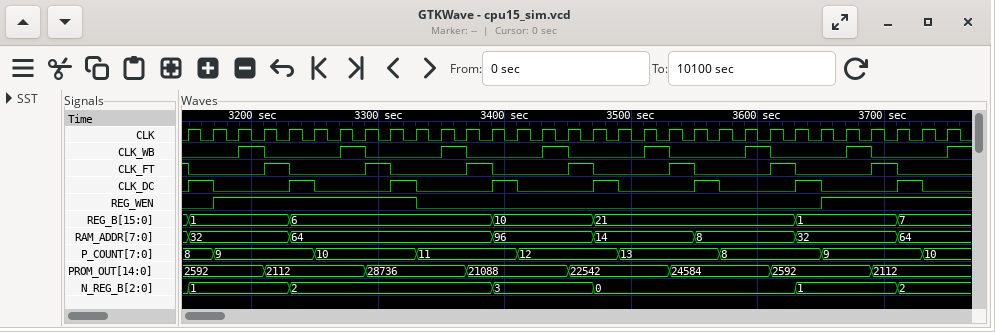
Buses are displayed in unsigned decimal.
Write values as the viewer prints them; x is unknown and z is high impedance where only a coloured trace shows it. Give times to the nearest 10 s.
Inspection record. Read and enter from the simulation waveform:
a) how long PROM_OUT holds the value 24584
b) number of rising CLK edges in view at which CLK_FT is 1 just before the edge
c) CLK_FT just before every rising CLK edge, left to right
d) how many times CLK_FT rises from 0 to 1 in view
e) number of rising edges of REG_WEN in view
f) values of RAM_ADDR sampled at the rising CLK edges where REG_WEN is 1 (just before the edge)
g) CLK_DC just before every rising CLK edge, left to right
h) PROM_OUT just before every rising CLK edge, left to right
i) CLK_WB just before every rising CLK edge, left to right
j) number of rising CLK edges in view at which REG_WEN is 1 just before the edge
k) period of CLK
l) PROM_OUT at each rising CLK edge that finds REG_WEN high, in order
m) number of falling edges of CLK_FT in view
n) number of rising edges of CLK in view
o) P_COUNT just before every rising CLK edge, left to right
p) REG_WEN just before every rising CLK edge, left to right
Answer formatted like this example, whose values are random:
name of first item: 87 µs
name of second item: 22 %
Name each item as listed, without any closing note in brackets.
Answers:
how long PROM_OUT holds the value 24584: 80 s
number of rising CLK edges in view at which CLK_FT is 1 just before the edge: 8
CLK_FT just before every rising CLK edge, left to right: 1 0 0 0 1 0 0 0 1 0 0 0 1 0 0 0 1 0 0 0 1 0 0 0 1 0 0 0 1 0 0
how many times CLK_FT rises from 0 to 1 in view: 7
number of rising edges of REG_WEN in view: 2
values of RAM_ADDR sampled at the rising CLK edges where REG_WEN is 1: 32, 32, 32, 64, 64, 64, 64, 64, 32, 32, 32, 64, 64
CLK_DC just before every rising CLK edge, left to right: 0 1 0 0 0 1 0 0 0 1 0 0 0 1 0 0 0 1 0 0 0 1 0 0 0 1 0 0 0 1 0
PROM_OUT just before every rising CLK edge, left to right: 2592, 2592, 2592, 2592, 2112, 2112, 2112, 2112, 28736, 28736, 28736, 28736, 21088, 21088, 21088, 21088, 22542, 22542, 22542, 22542, 24584, 24584, 24584, 24584, 2592, 2592, 2592, 2592, 2112, 2112, 2112
CLK_WB just before every rising CLK edge, left to right: 0 0 0 1 0 0 0 1 0 0 0 1 0 0 0 1 0 0 0 1 0 0 0 1 0 0 0 1 0 0 0
number of rising CLK edges in view at which REG_WEN is 1 just before the edge: 13
period of CLK: 20 s
PROM_OUT at each rising CLK edge that finds REG_WEN high, in order: 2592, 2592, 2112, 2112, 2112, 2112, 28736, 28736, 2592, 2592, 2112, 2112, 2112
number of falling edges of CLK_FT in view: 8
number of rising edges of CLK in view: 31
P_COUNT just before every rising CLK edge, left to right: 8, 8, 9, 9, 9, 9, 10, 10, 10, 10, 11, 11, 11, 11, 12, 12, 12, 12, 13, 13, 13, 13, 8, 8, 8, 8, 9, 9, 9, 9, 10
REG_WEN just before every rising CLK edge, left to right: 0 0 1 1 1 1 1 1 1 1 0 0 0 0 0 0 0 0 0 0 0 0 0 0 0 0 1 1 1 1 1
